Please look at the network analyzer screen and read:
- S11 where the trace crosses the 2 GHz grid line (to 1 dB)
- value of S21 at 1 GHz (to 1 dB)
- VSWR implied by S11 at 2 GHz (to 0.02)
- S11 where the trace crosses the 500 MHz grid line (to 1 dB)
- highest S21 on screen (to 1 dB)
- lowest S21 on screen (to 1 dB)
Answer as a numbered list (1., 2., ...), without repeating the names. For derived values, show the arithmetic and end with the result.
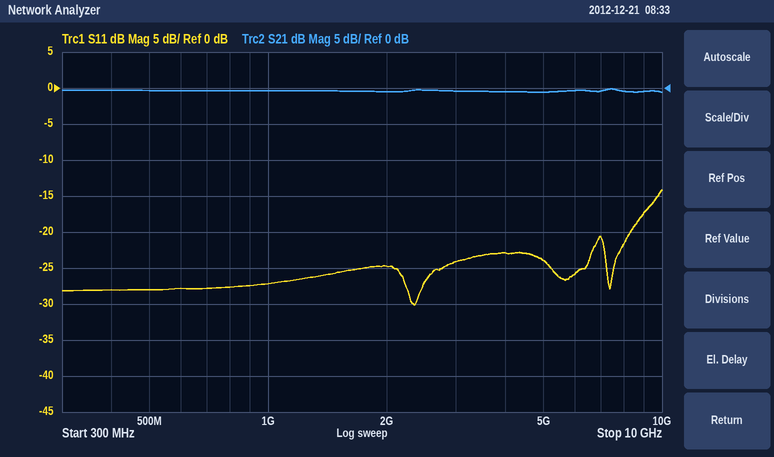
1. -25 dB
2. 0 dB
3. |Γ| = 10^(-25/20) = 0.0562; VSWR = (1 + 0.0562)/(1 − 0.0562) ≈ 1.12
4. -28 dB
5. 0 dB
6. -1 dB
